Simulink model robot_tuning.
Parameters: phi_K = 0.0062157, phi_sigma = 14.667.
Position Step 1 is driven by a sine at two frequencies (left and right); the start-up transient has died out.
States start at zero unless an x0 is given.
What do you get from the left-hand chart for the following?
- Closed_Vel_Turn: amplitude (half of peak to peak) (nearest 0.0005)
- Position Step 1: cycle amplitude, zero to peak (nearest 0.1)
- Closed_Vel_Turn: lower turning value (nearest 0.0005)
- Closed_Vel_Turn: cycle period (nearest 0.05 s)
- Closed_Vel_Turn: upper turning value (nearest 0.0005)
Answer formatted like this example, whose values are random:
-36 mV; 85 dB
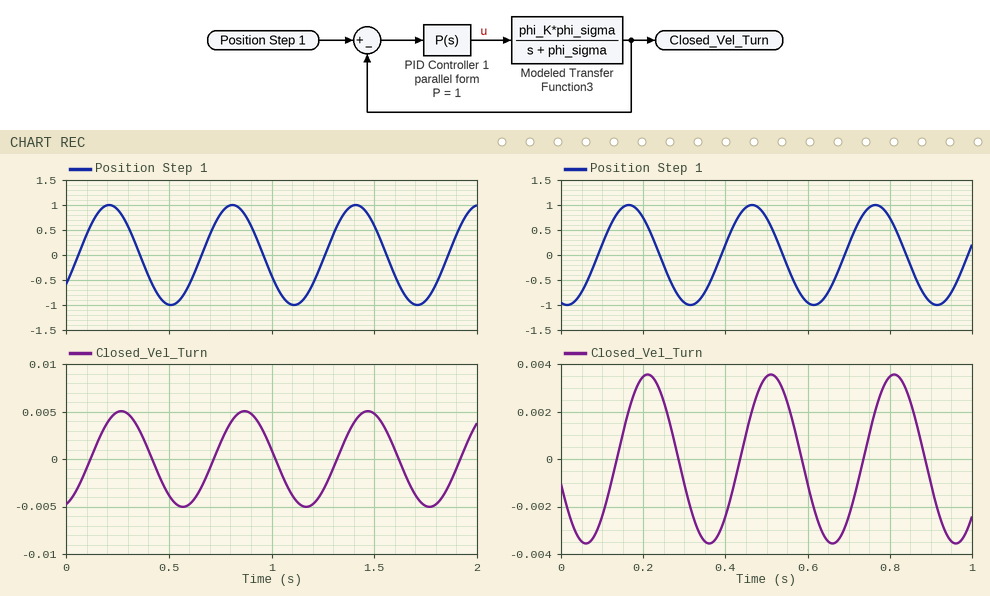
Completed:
0.0050; 1.0; -0.0050; 0.60 s; 0.0050
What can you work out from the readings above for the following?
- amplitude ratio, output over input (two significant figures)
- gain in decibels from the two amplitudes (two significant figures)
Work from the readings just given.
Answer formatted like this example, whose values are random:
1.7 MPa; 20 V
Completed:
0.0050; -46 dB
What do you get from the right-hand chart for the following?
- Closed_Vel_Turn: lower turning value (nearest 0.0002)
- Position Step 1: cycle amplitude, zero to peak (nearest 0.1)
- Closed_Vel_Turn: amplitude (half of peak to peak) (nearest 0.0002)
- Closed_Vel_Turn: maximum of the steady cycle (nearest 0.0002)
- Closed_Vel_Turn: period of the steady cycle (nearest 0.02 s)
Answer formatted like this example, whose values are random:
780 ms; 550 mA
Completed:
-0.0036; 1.0; 0.0036; 0.0036; 0.30 s
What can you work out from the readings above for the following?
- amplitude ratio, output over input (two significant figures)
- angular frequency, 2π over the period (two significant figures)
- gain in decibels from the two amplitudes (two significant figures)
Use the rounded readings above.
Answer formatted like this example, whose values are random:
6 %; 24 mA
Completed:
0.0036; 21 rad/s; -49 dB
